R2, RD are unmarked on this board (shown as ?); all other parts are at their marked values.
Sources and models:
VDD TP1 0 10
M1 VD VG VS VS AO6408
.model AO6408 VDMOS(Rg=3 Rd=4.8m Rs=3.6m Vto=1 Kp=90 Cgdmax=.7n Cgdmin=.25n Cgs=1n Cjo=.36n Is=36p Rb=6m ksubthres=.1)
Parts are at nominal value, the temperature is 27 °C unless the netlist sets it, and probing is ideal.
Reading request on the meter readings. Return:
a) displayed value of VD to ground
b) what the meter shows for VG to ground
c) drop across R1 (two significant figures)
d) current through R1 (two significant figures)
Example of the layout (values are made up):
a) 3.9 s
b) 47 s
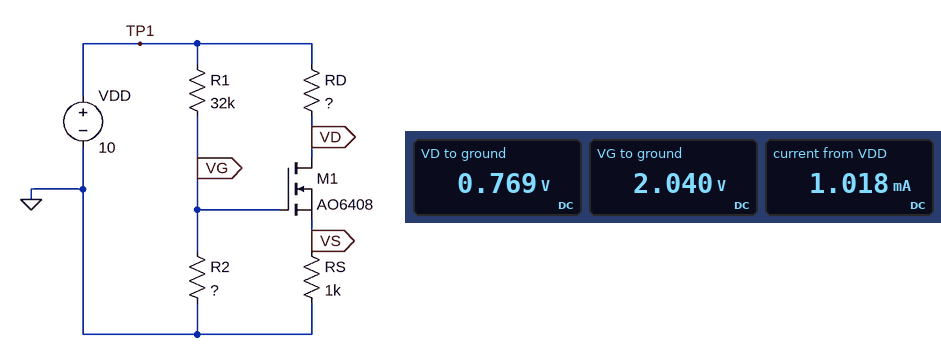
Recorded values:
a) 0.769 V
b) 2.040 V
c) 8.0 V
d) 250 µA
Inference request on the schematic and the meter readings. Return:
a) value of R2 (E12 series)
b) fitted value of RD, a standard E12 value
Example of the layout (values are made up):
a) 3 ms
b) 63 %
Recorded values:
a) 8.2 kΩ
b) 12 kΩ
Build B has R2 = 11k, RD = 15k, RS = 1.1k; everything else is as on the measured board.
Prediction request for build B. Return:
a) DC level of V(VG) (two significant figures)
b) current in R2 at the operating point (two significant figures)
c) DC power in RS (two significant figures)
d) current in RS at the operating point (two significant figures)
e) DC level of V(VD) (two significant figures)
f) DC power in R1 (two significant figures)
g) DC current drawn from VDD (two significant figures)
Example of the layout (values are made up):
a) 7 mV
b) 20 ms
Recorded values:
a) 2.6 V
b) 230 µA
c) 420 µW
d) 620 µA
e) 680 mV
f) 1.7 mW
g) 850 µA
